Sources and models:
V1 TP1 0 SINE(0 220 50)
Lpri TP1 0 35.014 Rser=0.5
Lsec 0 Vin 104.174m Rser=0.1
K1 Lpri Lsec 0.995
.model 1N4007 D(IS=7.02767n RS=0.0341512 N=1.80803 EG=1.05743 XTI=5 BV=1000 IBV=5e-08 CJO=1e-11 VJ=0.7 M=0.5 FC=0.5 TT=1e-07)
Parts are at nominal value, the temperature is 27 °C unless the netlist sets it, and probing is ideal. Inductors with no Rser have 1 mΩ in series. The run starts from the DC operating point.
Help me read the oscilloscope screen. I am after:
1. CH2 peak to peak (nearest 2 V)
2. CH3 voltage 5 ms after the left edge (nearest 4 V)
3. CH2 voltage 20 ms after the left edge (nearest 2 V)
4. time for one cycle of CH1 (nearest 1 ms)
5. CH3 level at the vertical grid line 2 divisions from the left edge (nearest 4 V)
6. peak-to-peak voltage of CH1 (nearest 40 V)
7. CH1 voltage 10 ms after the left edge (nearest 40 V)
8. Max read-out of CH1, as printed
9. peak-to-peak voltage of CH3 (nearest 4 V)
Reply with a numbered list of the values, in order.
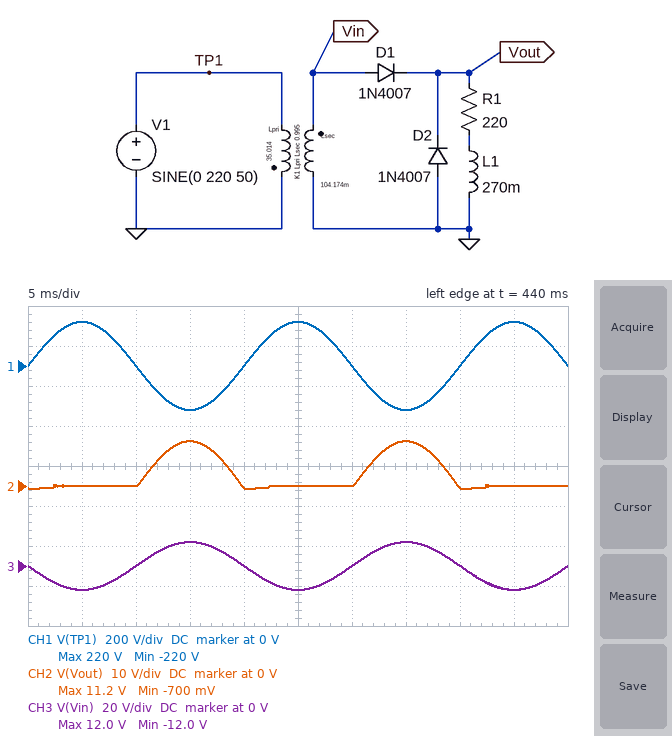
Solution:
1. 12 V
2. -12 V
3. 0 V
4. 20 ms
5. 0 V
6. 440 V
7. 0 V
8. 220 V
9. 24 V
